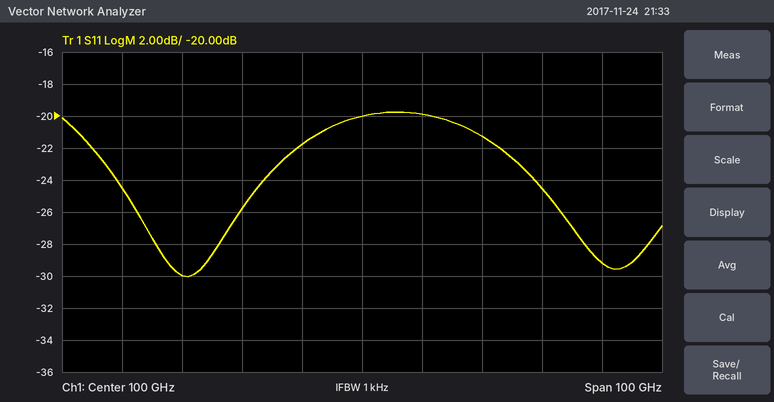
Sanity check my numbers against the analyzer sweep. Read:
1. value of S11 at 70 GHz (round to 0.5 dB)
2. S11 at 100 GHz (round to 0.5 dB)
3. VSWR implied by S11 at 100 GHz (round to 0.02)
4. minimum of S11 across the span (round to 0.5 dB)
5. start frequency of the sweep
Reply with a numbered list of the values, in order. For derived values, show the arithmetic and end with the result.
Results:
1. -30.0 dB
2. -20.0 dB
3. |Γ| = 10^(-20/20) = 0.1000; VSWR = (1 + 0.1000)/(1 − 0.1000) ≈ 1.22
4. -30.0 dB
5. 50 GHz
